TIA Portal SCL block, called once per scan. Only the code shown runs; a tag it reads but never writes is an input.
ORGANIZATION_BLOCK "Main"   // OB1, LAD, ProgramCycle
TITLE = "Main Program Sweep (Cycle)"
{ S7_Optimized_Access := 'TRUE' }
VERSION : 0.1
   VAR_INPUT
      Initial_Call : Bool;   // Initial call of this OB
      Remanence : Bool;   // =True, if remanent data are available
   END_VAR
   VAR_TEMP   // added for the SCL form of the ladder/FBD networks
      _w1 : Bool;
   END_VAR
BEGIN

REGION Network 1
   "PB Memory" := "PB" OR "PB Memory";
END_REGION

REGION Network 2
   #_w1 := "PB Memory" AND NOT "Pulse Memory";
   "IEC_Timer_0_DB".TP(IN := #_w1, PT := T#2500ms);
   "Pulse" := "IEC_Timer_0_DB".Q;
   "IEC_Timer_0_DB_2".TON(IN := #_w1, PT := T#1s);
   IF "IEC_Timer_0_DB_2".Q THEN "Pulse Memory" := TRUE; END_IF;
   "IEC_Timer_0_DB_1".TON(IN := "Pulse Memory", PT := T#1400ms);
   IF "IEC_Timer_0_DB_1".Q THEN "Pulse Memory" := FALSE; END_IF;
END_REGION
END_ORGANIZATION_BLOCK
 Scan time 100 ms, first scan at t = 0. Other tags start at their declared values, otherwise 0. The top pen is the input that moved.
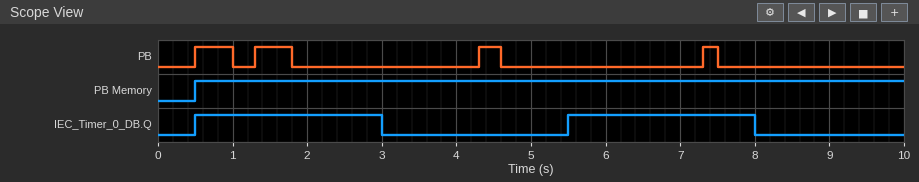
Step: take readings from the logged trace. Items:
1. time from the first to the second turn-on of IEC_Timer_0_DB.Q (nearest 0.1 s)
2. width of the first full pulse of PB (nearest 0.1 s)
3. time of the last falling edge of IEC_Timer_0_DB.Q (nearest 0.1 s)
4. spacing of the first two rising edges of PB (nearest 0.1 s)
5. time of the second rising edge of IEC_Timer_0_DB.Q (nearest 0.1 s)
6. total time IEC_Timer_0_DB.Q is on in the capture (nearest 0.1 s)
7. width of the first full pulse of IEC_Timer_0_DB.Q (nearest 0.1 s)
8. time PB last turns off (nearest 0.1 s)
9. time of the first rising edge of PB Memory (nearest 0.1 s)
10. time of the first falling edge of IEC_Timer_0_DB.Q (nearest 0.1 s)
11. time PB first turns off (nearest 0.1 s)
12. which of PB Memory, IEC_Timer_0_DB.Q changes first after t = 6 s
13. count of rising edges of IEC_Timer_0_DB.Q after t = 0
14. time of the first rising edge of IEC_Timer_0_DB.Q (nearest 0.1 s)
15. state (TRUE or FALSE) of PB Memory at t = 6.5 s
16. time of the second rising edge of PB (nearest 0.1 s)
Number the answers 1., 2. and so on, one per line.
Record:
1. 5.0 s
2. 0.5 s
3. 8.0 s
4. 0.8 s
5. 5.5 s
6. 5.0 s
7. 2.5 s
8. 7.5 s
9. 0.5 s
10. 3.0 s
11. 1.0 s
12. IEC_Timer_0_DB.Q
13. 2
14. 0.5 s
15. TRUE
16. 1.3 s
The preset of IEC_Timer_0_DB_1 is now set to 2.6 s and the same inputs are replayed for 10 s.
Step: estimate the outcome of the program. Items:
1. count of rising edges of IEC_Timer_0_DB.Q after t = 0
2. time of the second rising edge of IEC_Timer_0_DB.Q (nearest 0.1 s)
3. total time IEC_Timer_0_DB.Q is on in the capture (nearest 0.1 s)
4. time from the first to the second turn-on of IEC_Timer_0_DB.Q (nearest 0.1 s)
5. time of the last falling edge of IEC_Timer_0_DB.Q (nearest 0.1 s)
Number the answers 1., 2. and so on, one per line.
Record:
1. 3
2. 4.2 s
3. 7.1 s
4. 3.7 s
5. 6.7 s
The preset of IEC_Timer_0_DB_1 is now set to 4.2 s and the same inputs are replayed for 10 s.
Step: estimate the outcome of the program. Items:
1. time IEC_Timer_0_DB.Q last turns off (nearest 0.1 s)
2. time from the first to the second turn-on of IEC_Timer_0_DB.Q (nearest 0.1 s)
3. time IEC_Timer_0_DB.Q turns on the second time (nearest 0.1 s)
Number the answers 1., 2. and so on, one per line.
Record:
1. 8.3 s
2. 5.3 s
3. 5.8 s
